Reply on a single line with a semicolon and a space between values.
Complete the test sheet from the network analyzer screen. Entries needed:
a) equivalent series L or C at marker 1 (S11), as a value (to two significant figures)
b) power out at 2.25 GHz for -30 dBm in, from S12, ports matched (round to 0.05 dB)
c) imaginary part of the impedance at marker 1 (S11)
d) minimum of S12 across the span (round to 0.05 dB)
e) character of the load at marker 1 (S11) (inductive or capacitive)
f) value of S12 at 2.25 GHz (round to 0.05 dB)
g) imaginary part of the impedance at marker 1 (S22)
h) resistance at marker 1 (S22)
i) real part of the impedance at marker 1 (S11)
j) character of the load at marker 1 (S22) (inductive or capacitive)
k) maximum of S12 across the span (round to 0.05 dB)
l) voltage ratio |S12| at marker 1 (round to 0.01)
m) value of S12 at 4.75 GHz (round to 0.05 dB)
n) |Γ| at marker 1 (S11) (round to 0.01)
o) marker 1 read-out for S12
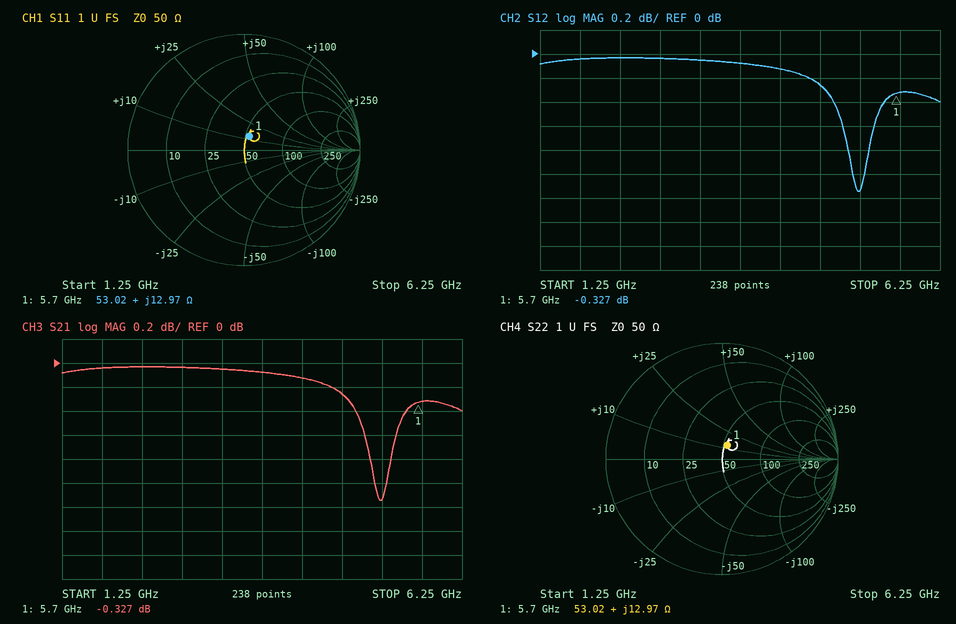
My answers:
360 pH; -30.05 dBm; +12.97 Ω; -1.15 dB; inductive; -0.05 dB; +12.97 Ω; 53.02 Ω; 53.02 Ω; inductive; -0.05 dB; 0.96; -0.25 dB; 0.13; -0.327 dB
